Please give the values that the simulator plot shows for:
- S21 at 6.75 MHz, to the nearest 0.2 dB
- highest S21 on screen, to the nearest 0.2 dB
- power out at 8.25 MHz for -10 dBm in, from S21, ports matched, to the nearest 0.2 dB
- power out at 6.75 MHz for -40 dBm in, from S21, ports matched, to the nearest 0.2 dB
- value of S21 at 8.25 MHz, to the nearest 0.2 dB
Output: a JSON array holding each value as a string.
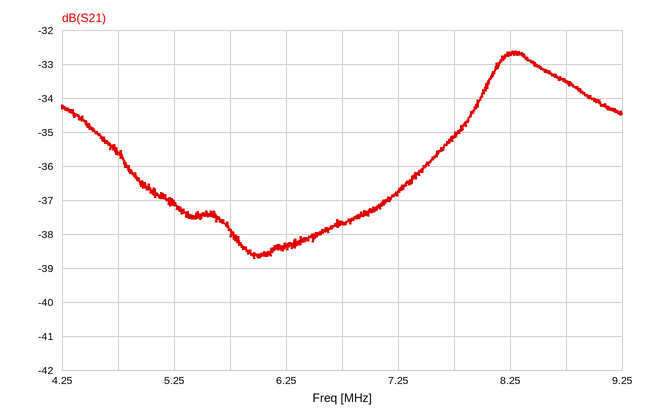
["-37.6 dB", "-32.6 dB", "-42.6 dBm", "-77.6 dBm", "-32.6 dB"]
